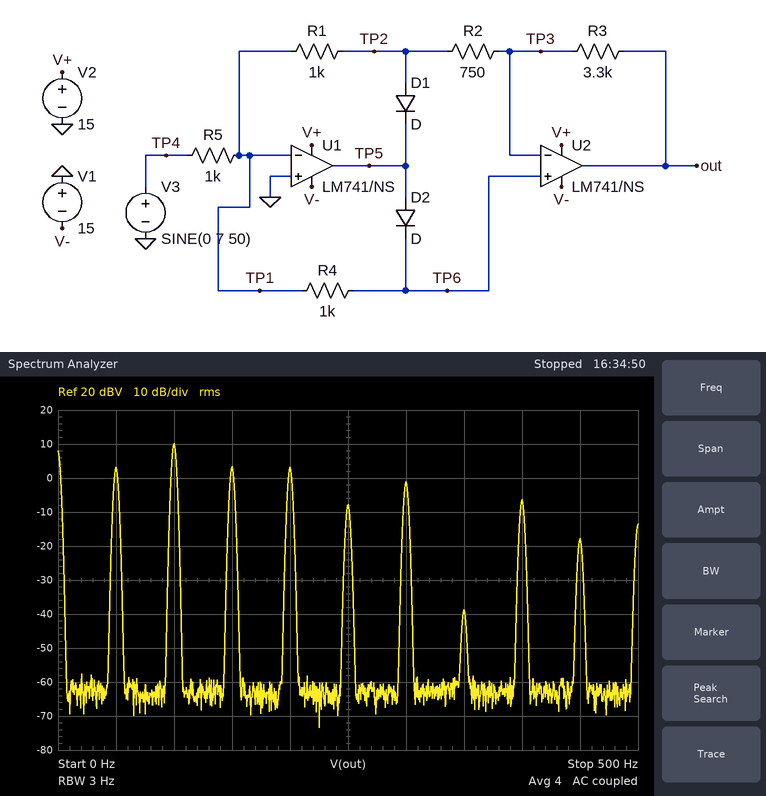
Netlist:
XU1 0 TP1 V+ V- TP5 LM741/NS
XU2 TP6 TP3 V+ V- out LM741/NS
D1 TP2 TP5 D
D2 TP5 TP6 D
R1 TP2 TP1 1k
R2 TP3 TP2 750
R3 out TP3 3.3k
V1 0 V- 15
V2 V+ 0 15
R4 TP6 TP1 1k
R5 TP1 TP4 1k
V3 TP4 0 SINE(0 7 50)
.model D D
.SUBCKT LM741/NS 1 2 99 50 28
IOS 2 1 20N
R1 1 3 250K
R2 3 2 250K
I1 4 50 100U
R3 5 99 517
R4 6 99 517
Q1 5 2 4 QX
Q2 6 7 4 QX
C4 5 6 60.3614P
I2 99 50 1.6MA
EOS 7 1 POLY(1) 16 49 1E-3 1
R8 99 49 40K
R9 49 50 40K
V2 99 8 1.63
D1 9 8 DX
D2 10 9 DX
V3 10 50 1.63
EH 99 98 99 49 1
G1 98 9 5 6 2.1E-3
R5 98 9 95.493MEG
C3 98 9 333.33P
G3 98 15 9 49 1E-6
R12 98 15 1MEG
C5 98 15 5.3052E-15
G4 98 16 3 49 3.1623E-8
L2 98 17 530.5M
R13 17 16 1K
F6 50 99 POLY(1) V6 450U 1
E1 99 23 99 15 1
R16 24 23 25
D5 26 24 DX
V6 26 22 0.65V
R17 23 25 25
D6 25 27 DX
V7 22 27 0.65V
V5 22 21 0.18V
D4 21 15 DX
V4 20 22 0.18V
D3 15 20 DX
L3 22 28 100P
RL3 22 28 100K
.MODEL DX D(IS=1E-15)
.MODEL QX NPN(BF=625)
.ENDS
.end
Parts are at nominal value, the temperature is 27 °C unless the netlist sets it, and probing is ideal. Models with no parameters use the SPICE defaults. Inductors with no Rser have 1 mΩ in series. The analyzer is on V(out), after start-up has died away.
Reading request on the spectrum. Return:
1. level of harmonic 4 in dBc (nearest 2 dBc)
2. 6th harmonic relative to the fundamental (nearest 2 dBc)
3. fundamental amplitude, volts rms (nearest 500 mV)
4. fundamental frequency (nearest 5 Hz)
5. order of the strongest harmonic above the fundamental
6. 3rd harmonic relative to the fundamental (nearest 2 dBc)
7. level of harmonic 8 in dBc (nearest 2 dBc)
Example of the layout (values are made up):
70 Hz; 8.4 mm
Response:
0 dBc; -4 dBc; 1.5 V; 50 Hz; 2; 0 dBc; -10 dBc
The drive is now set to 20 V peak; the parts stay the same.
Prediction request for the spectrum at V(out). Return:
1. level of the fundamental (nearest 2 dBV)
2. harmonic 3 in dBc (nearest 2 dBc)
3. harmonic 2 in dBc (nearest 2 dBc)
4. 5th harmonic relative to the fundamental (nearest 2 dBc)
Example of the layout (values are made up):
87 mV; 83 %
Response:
-22 dBV; 12 dBc; 26 dBc; 16 dBc
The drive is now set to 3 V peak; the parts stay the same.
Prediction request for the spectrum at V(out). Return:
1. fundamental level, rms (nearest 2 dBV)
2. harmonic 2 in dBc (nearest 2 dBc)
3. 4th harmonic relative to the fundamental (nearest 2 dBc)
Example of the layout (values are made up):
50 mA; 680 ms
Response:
8 dBV; 0 dBc; -14 dBc
